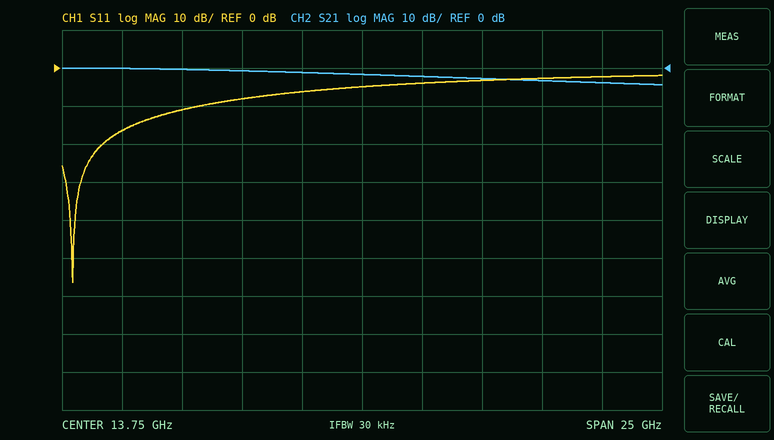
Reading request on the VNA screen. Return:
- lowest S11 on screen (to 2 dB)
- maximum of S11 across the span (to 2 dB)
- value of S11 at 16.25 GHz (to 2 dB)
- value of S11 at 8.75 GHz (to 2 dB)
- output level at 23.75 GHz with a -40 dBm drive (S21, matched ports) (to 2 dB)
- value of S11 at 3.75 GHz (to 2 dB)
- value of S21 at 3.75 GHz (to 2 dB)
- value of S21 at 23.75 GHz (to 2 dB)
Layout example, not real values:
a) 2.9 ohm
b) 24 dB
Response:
a) -56 dB
b) -2 dB
c) -4 dB
d) -8 dB
e) -44 dBm
f) -16 dB
g) 0 dB
h) -4 dB
